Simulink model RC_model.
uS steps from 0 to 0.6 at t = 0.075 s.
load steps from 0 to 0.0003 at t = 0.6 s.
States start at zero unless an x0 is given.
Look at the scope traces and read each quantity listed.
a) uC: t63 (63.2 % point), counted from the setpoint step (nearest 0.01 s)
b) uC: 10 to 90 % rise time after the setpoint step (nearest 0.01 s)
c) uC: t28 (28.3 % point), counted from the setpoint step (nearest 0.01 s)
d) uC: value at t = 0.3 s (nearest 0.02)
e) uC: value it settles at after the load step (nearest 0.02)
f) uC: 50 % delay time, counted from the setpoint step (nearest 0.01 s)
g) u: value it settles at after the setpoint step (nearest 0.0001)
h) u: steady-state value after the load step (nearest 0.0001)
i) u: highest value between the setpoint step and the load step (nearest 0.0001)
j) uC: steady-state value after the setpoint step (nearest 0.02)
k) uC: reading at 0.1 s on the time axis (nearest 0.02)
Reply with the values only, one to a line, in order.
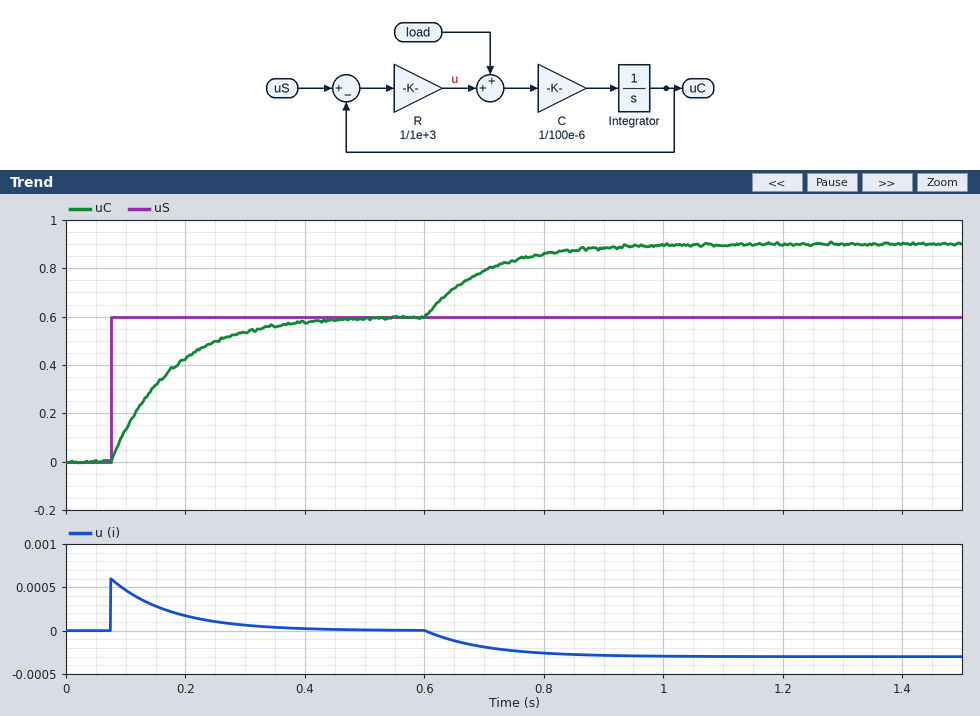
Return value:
0.10 s
0.22 s
0.03 s
0.54
0.90
0.07 s
0.0000
-0.0003
0.0006
0.60
0.14
